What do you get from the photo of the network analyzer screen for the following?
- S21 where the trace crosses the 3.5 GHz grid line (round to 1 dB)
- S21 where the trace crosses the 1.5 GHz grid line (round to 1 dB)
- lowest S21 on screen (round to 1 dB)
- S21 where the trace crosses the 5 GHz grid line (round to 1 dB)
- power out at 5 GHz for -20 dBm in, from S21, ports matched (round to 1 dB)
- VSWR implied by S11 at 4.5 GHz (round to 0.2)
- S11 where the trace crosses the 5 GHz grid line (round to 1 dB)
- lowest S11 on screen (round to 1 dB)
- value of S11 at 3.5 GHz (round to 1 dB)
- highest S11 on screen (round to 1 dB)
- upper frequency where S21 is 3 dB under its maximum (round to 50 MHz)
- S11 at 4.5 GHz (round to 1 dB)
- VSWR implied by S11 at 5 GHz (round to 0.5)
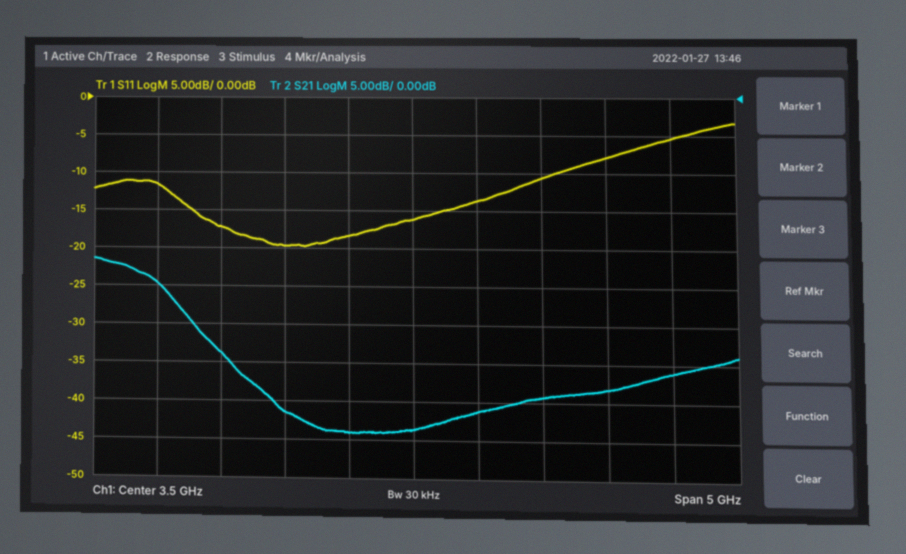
-44 dB
-25 dB
-44 dB
-38 dB
-58 dBm
1.8
-8 dB
-20 dB
-16 dB
-3 dB
1.50 GHz
-11 dB
2.5
